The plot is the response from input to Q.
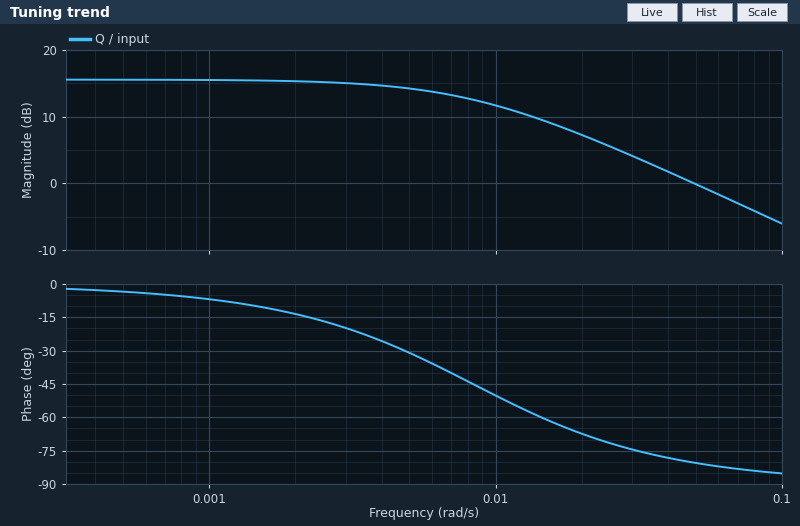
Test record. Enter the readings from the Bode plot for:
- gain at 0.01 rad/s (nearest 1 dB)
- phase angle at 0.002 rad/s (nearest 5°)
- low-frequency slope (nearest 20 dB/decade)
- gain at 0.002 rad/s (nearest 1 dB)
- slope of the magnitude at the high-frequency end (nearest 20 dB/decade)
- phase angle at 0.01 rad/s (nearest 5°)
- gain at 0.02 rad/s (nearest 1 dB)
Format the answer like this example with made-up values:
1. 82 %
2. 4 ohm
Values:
1. 12 dB
2. -15°
3. 0 dB/decade
4. 15 dB
5. -20 dB/decade
6. -50°
7. 7 dB
